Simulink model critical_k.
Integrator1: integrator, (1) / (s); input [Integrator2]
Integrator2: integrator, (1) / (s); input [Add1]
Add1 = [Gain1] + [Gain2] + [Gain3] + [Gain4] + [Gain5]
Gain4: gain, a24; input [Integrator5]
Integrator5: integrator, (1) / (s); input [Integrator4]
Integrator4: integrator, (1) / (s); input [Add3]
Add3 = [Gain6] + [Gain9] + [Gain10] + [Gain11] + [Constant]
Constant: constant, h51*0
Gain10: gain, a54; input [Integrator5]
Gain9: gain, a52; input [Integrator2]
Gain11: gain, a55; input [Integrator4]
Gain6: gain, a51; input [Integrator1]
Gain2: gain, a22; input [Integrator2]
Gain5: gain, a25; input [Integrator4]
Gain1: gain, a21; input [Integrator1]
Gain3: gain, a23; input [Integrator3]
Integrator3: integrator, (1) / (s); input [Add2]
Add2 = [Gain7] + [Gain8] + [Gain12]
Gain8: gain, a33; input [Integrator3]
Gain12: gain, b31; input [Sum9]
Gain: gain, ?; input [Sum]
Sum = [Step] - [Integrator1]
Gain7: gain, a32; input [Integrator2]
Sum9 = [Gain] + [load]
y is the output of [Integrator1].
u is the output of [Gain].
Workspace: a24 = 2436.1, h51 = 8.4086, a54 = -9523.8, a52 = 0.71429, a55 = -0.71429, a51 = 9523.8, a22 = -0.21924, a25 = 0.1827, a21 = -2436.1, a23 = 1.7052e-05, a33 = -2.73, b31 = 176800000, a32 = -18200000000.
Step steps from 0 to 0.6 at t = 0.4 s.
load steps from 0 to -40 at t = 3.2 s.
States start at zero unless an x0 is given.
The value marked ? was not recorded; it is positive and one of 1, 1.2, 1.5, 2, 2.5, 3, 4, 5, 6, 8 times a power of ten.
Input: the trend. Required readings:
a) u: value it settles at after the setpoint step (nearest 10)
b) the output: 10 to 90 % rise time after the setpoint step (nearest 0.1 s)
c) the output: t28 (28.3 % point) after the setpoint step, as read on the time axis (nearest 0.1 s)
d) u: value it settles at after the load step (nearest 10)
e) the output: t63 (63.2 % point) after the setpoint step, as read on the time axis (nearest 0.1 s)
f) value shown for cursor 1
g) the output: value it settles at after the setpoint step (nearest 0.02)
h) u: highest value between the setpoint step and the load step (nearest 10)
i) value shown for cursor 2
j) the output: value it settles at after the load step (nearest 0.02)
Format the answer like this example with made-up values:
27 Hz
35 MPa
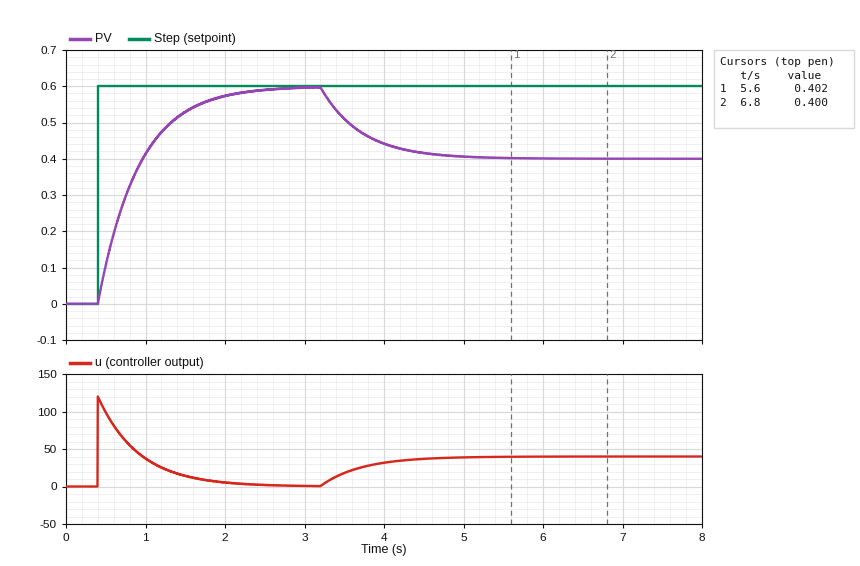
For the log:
0
1.1 s
0.6 s
40
0.9 s
0.402
0.60
120
0.400
0.40
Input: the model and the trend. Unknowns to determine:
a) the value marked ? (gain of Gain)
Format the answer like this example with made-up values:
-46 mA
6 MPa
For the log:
200
